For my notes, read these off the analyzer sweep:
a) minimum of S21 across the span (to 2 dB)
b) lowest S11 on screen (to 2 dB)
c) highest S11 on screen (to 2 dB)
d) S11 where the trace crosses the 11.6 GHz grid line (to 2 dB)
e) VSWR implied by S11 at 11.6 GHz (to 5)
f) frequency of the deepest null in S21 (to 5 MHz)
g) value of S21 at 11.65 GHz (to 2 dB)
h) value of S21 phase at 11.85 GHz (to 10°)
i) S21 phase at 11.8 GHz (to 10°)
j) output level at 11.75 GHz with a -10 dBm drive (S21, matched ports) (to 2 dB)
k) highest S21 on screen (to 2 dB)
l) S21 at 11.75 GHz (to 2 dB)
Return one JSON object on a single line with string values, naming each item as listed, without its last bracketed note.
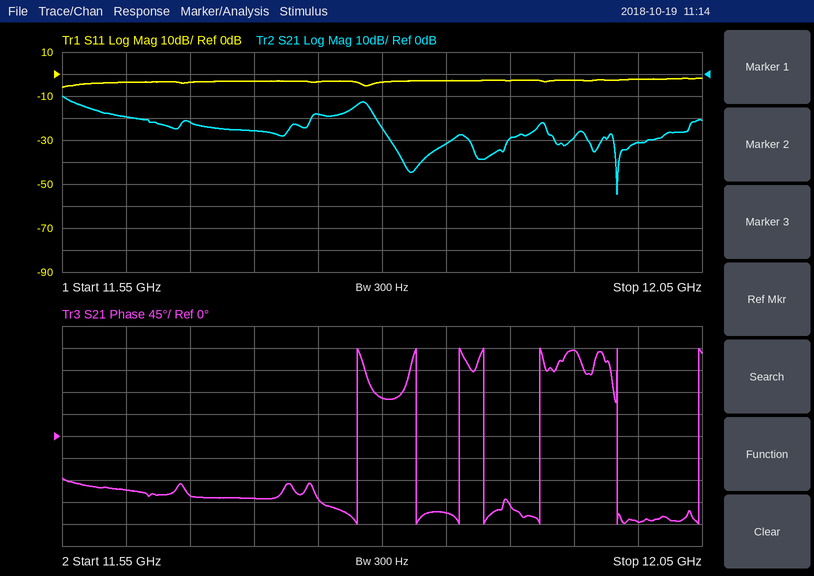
{"minimum of S21 across the span": "-54 dB", "lowest S11 on screen": "-6 dB", "highest S11 on screen": "-2 dB", "S11 where the trace crosses the 11.6 GHz grid line": "-4 dB", "VSWR implied by S11 at 11.6 GHz": "5", "frequency of the deepest null in S21": "11.985 GHz", "value of S21 at 11.65 GHz": "-22 dB", "value of S21 phase at 11.85 GHz": "-160°", "S21 phase at 11.8 GHz": "80°", "output level at 11.75 GHz with a -10 dBm drive (S21, matched ports)": "-28 dBm", "highest S21 on screen": "-10 dB", "S21 at 11.75 GHz": "-18 dB"}
